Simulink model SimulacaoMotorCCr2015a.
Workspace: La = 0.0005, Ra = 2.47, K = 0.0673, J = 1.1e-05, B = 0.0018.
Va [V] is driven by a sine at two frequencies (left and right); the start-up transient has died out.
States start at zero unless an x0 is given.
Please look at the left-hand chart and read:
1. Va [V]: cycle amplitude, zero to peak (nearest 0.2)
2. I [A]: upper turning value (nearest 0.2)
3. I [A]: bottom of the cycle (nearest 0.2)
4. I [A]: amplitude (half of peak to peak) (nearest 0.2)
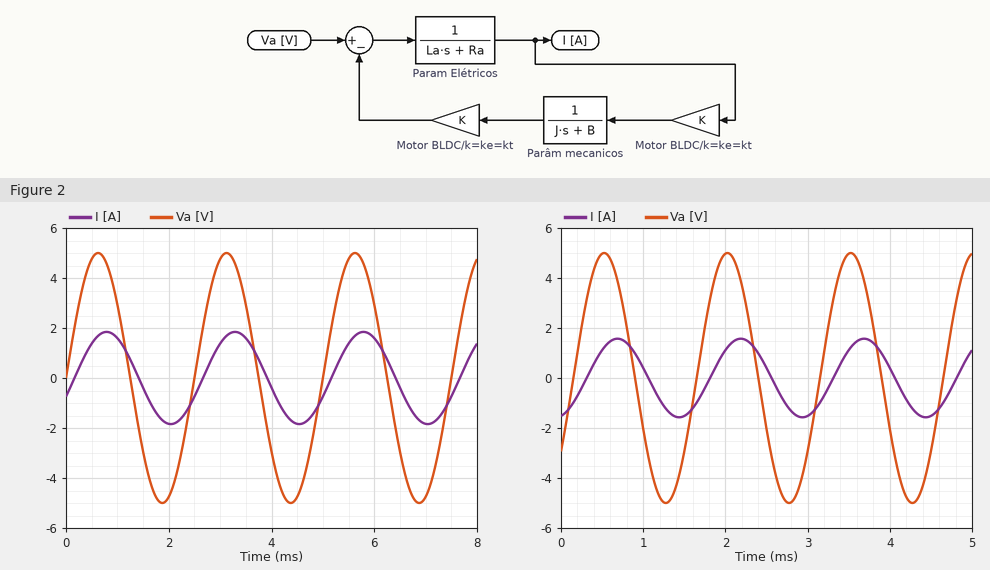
5.0
1.8
-1.8
1.8
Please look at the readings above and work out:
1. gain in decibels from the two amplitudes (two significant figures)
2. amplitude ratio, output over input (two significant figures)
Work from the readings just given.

-8.9 dB
0.36
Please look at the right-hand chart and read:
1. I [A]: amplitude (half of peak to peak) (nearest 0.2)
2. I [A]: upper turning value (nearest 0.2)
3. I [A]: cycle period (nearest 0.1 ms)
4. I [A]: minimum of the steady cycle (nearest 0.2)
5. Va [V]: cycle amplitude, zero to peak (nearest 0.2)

1.6
1.6
1.5 ms
-1.6
5.0
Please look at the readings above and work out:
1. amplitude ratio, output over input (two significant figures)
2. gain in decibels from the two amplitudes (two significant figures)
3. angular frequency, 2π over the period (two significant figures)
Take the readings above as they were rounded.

0.32
-9.9 dB
4.2 rad/ms
